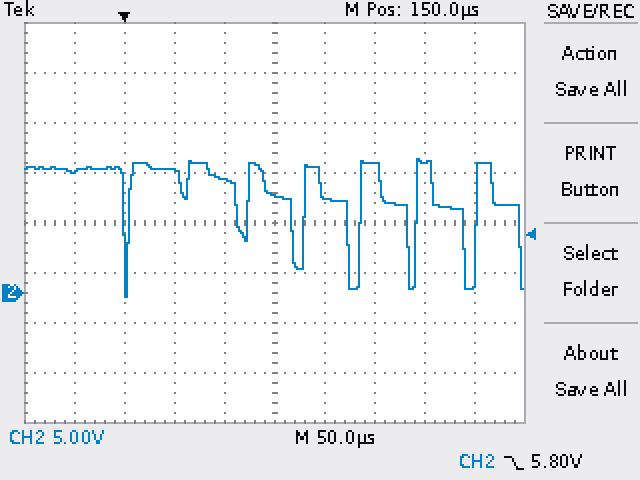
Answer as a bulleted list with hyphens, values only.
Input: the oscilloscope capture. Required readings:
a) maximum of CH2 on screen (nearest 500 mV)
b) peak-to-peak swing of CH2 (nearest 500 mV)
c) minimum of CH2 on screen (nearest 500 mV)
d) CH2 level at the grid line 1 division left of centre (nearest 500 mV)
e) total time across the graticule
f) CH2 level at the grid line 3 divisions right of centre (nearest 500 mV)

- 13.5 V
- 14.0 V
- -500 mV
- 11.5 V
- 500 µs
- 13.0 V
